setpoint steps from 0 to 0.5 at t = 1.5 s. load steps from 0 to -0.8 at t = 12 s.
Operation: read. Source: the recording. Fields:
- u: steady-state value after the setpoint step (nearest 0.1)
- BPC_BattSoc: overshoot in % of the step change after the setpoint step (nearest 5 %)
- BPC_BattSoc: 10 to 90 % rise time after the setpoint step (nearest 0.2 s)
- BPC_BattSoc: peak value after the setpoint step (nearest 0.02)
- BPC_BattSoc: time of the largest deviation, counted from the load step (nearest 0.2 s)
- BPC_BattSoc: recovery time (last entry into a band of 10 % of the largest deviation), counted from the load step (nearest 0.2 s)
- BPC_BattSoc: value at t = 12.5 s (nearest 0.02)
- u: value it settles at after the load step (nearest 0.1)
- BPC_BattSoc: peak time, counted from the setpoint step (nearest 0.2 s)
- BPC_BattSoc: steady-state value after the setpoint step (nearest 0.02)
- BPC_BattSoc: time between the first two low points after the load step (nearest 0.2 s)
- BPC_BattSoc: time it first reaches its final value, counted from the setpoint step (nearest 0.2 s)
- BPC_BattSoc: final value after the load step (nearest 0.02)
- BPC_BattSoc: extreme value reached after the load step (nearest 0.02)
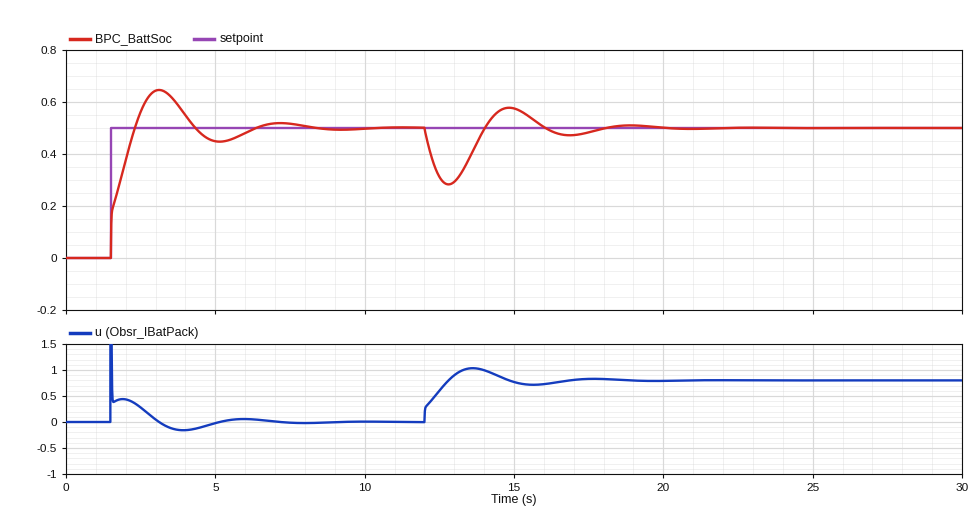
0.0
30 %
0.6 s
0.64
0.8 s
5.4 s
0.32
0.8
1.6 s
0.50
4.0 s
0.8 s
0.50
0.28
